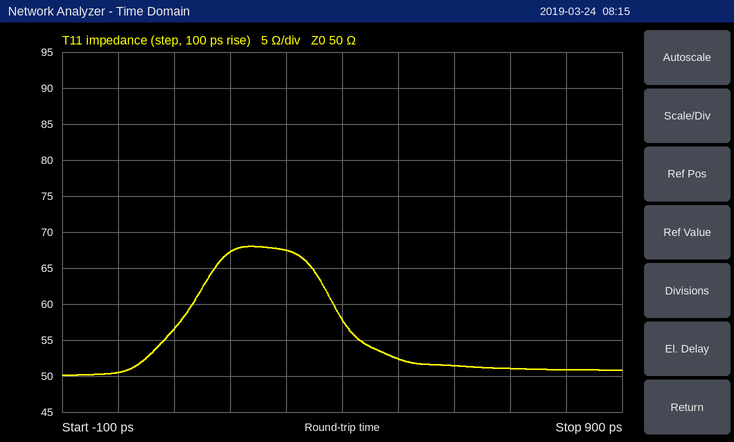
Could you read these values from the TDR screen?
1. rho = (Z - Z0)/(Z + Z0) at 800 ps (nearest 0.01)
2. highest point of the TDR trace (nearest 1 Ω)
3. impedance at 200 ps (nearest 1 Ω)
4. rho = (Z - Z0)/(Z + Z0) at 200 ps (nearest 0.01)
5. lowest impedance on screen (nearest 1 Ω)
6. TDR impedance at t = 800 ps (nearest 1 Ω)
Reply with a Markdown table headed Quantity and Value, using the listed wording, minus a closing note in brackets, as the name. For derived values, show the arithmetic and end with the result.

| Quantity | Value |
|---|---|
| rho = (Z - Z0)/(Z + Z0) at 800 ps | (51 − 50)/(51 + 50) ≈ +0.01 |
| highest point of the TDR trace | 68 Ω |
| impedance at 200 ps | 67 Ω |
| rho = (Z - Z0)/(Z + Z0) at 200 ps | (67 − 50)/(67 + 50) ≈ +0.15 |
| lowest impedance on screen | 50 Ω |
| TDR impedance at t = 800 ps | 51 Ω |
